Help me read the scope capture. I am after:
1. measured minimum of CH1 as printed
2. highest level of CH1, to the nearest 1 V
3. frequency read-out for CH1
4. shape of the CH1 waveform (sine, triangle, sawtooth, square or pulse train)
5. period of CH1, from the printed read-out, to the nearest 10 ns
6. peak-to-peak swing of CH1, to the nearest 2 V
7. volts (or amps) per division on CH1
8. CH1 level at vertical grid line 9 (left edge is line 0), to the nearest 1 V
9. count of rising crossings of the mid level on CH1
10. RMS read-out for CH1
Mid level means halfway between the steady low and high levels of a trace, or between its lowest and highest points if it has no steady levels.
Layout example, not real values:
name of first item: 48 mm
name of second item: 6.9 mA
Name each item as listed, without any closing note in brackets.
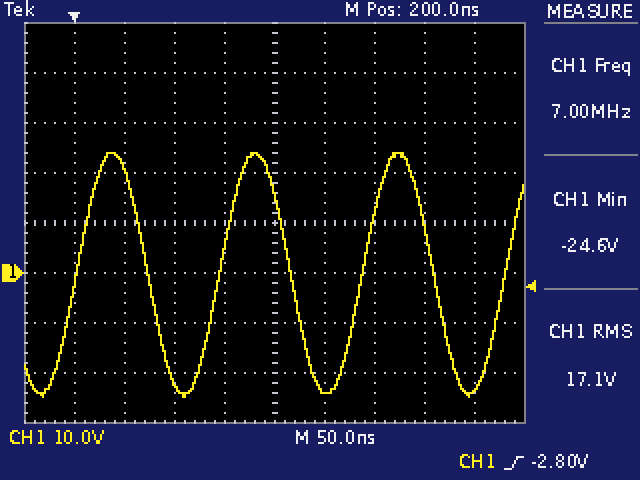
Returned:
measured minimum of CH1 as printed: -24.6 V
highest level of CH1, to the nearest 1 V: 24 V
frequency read-out for CH1: 7.00 MHz
shape of the CH1 waveform: sine
period of CH1, from the printed read-out, to the nearest 10 ns: 140 ns
peak-to-peak swing of CH1, to the nearest 2 V: 48 V
volts (or amps) per division on CH1: 10 V
CH1 level at vertical grid line 9 (left edge is line 0), to the nearest 1 V: -23 V
count of rising crossings of the mid level on CH1: 4
RMS read-out for CH1: 17.1 V
